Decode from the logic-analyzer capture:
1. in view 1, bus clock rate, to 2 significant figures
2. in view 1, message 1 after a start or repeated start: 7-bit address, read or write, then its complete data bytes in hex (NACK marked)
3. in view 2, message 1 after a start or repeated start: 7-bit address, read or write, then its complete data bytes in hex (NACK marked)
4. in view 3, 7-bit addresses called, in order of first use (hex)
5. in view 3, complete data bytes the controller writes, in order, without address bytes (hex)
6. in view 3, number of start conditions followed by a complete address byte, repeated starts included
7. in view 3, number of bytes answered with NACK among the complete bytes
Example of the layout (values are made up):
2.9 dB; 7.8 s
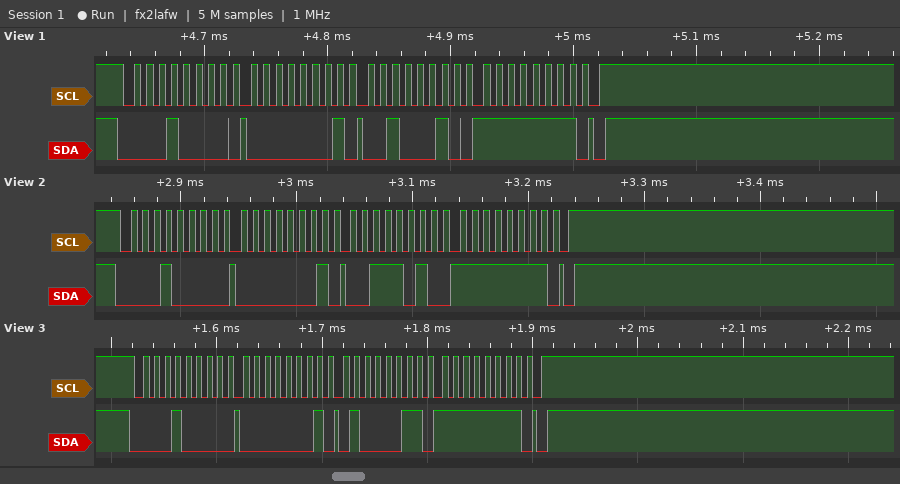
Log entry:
100 kHz; 0x08 write: 01 22 FF; 0x08 write: 01 3A FF; 0x08; 01 43 FF; 1; 0
